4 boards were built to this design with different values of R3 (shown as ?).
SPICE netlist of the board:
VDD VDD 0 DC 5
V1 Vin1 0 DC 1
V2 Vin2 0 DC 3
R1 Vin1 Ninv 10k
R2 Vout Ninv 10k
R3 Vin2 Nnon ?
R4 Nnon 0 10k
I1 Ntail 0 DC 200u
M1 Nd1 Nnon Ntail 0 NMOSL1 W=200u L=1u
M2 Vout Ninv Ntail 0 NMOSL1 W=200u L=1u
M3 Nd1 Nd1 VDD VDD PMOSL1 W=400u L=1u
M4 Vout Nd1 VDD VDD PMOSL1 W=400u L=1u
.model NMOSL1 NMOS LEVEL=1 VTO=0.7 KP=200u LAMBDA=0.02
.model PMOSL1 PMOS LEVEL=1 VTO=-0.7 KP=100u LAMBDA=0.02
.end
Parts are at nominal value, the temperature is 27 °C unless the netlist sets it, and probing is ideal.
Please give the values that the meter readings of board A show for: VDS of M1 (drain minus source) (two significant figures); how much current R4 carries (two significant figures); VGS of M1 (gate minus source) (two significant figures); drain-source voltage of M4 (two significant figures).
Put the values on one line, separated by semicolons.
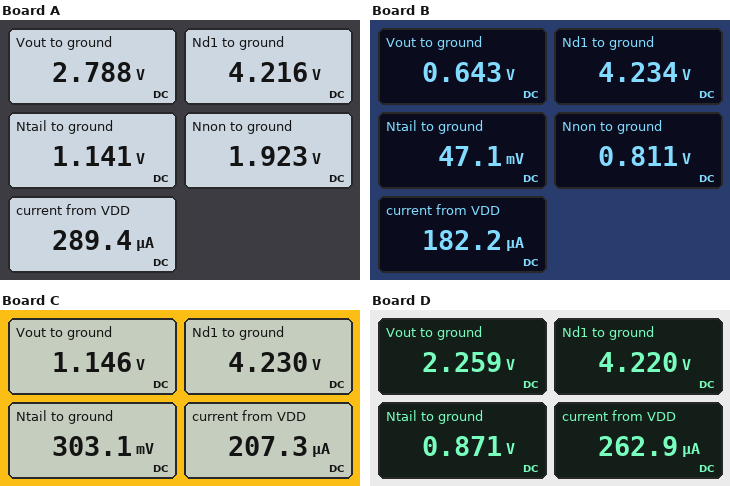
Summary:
3.1 V; 190 µA; 780 mV; -2.2 V
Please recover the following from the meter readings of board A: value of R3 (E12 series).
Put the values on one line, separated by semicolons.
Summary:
5.6 kΩ
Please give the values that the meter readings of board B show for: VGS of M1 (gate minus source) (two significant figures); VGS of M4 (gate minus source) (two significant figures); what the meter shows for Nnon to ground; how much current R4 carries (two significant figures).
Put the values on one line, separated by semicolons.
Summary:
760 mV; -770 mV; 0.811 V; 81 µA
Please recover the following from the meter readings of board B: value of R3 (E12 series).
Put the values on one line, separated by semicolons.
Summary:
27 kΩ
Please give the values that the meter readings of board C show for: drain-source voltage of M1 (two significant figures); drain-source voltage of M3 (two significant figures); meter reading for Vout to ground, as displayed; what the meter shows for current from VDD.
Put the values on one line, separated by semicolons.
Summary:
3.9 V; -770 mV; 1.146 V; 207.3 µA
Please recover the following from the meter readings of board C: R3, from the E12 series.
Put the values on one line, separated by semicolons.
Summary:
18 kΩ
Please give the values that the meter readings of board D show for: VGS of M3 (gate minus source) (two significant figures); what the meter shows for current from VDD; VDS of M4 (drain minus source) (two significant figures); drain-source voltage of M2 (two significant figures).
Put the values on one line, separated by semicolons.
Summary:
-780 mV; 262.9 µA; -2.7 V; 1.4 V
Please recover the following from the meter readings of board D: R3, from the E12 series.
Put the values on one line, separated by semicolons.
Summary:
8.2 kΩ
